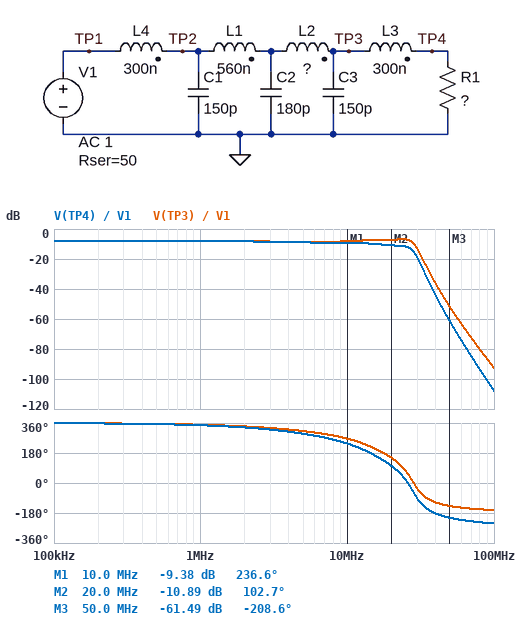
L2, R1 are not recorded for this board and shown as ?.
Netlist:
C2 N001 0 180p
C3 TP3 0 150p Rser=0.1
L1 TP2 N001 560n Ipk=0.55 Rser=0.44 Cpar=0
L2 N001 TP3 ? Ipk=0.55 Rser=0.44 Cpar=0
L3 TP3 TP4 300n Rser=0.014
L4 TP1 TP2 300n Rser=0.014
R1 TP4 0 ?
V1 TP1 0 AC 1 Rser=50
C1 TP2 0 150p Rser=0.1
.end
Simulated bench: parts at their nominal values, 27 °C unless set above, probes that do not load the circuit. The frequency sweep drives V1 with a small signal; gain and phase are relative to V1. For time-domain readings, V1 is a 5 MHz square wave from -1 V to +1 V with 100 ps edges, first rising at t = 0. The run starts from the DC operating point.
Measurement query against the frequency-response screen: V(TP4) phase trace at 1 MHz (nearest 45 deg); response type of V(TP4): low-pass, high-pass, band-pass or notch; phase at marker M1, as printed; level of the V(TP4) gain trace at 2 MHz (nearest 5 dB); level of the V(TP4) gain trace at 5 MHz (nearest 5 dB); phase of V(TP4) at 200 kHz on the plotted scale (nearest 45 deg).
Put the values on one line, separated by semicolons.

360 deg; low-pass; 236.6 deg; -10 dB; -10 dB; 360 deg
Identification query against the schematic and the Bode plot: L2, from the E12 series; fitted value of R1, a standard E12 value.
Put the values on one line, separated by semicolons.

1.2 µH; 33 Ω
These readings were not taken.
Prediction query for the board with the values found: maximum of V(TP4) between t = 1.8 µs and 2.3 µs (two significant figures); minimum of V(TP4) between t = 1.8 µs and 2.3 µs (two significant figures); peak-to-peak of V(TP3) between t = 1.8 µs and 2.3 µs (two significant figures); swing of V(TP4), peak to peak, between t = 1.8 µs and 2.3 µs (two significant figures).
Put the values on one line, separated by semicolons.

420 mV; -420 mV; 1.1 V; 840 mV
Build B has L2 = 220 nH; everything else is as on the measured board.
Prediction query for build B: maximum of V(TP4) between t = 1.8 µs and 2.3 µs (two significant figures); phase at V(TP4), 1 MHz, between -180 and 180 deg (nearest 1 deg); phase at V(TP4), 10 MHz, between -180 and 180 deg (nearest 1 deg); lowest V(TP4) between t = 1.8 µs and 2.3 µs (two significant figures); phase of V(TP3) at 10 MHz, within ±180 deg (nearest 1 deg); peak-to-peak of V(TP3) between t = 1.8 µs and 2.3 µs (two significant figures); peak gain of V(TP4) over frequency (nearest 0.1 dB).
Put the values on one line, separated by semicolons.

490 mV; -9 deg; -93 deg; -490 mV; -64 deg; 1.4 V; -7.9 dB
